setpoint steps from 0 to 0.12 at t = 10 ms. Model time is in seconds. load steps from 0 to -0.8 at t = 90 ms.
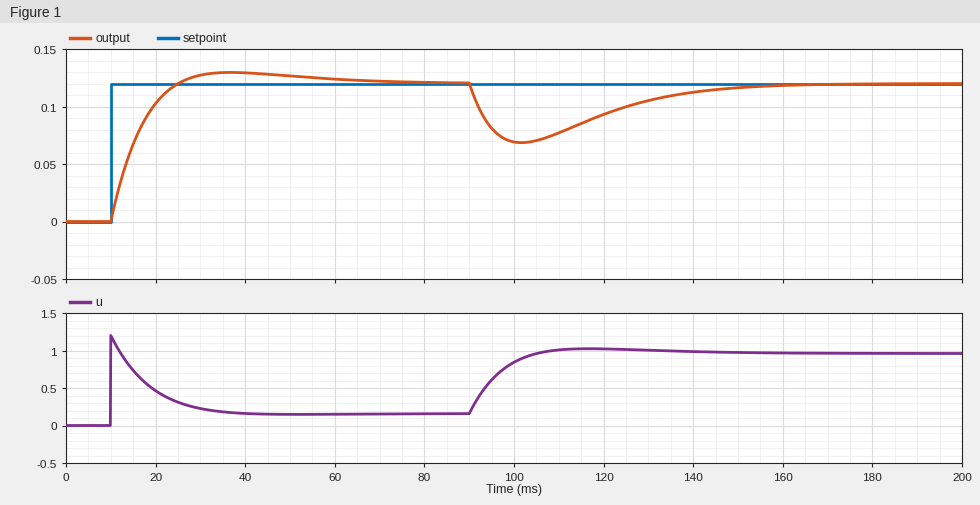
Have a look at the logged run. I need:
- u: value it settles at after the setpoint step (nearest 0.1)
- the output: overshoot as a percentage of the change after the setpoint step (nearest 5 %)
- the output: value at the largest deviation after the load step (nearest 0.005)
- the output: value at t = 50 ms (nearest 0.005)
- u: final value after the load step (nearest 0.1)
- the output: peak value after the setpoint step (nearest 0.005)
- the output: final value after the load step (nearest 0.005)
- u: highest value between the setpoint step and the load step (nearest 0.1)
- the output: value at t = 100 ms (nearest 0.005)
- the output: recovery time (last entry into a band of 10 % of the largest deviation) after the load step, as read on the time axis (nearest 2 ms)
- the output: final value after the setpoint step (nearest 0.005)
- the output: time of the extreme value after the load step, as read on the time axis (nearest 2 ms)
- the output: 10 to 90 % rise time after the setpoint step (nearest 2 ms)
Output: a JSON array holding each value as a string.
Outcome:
["0.2", "10 %", "0.070", "0.125", "1.0", "0.130", "0.120", "1.2", "0.070", "146 ms", "0.120", "102 ms", "10 ms"]
